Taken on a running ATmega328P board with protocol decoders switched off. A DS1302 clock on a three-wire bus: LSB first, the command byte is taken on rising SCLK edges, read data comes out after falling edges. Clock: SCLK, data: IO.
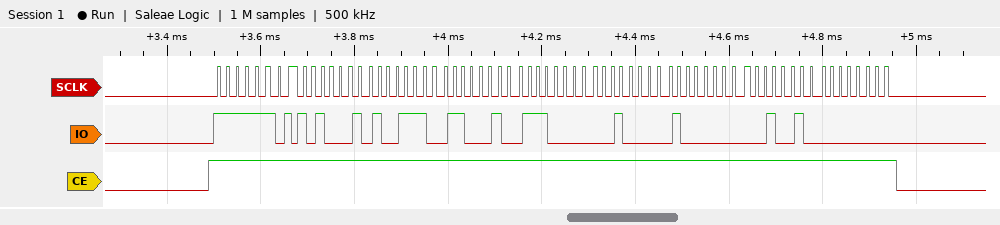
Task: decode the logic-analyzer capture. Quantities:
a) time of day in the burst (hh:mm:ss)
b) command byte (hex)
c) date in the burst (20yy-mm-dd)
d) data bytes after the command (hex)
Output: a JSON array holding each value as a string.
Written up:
["23:39:45", "0xBF", "2024-04-07", "45 39 23 07 04 01 24 00"]
